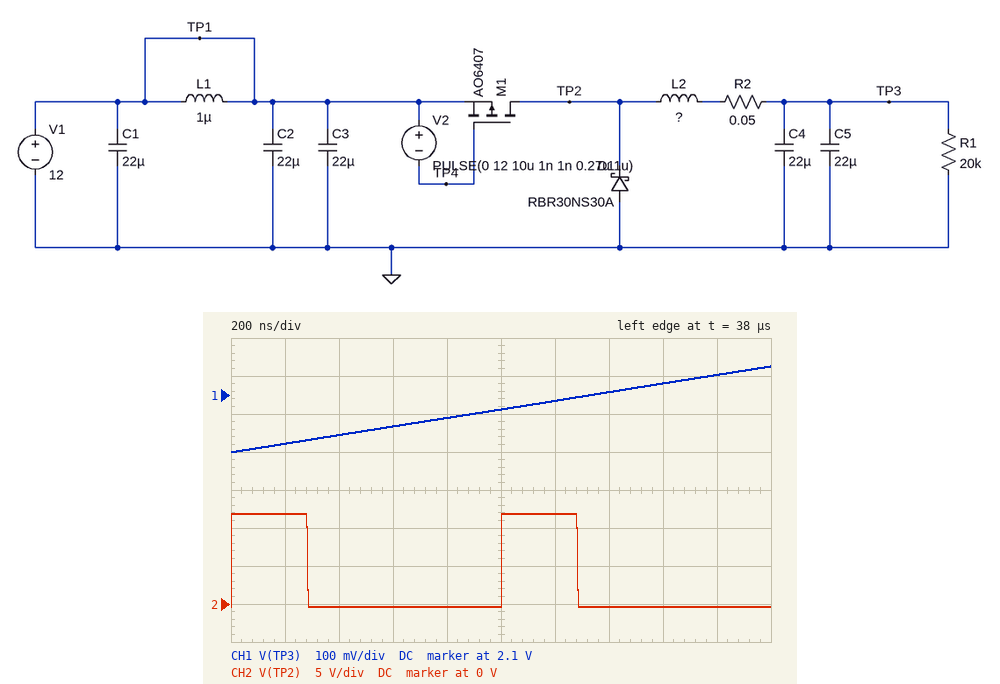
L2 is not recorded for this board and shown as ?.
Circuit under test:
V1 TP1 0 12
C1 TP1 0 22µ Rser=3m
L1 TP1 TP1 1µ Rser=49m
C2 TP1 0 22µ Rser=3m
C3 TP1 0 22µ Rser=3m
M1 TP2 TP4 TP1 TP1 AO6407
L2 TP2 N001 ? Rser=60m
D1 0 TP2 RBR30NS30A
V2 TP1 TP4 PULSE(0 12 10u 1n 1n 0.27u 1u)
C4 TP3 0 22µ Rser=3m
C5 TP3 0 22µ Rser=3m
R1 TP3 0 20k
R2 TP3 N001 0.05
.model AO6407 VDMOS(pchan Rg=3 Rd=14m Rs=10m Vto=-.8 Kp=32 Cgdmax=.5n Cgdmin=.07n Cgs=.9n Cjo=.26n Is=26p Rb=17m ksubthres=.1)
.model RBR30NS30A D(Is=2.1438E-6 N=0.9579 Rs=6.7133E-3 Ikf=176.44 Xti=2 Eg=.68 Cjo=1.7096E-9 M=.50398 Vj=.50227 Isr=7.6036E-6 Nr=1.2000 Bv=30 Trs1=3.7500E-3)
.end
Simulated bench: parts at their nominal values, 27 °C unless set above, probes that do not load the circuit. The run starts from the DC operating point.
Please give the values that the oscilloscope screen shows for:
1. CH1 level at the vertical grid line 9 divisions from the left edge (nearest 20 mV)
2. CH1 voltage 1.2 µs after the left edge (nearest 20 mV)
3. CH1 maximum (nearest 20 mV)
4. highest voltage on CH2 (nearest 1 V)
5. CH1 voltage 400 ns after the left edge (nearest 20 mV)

2.16 V
2.08 V
2.18 V
12 V
2.00 V
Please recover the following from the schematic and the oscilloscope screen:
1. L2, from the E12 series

12 µH
